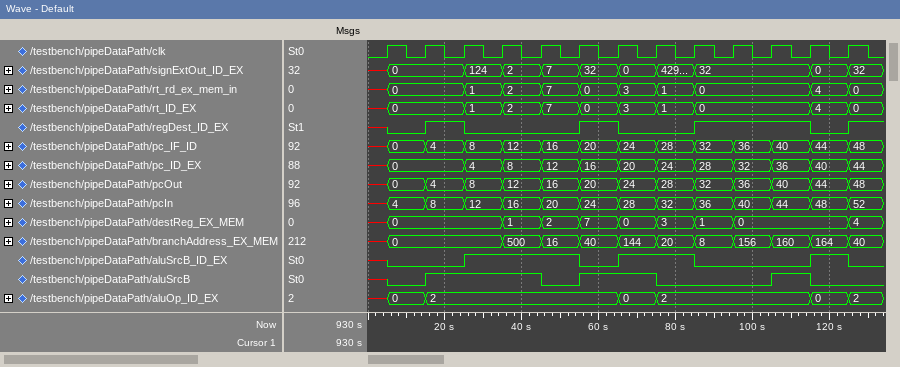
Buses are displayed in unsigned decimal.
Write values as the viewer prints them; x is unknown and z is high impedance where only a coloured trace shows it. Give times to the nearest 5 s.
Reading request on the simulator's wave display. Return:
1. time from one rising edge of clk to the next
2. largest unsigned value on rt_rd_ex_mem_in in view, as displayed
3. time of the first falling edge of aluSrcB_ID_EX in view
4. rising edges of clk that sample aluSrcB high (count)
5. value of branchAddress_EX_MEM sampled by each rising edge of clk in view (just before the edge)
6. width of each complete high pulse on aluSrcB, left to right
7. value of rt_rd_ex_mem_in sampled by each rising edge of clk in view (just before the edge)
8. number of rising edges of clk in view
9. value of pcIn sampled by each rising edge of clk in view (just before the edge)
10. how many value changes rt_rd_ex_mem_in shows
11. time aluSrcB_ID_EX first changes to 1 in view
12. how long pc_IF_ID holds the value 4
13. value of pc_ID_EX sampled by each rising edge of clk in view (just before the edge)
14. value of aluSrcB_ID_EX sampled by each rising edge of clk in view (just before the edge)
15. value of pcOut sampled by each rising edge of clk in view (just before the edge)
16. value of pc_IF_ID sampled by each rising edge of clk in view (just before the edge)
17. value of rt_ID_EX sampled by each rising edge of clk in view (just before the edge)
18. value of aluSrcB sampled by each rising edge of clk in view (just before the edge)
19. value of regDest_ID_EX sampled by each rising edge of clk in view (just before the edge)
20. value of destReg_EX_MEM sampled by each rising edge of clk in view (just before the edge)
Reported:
10 s
7
55 s
6
x, 0, 0, 0, 500, 16, 40, 144, 20, 8, 156, 160, 164
30 s, 20 s, 10 s
x, 0, 0, 1, 2, 7, 0, 3, 1, 0, 0, 0, 4
13
x, 4, 8, 12, 16, 20, 24, 28, 32, 36, 40, 44, 48
10
25 s
10 s
x, 0, 0, 4, 8, 12, 16, 20, 24, 28, 32, 36, 40
x 0 0 1 1 1 0 1 1 0 0 0 1
x, 0, 4, 8, 12, 16, 20, 24, 28, 32, 36, 40, 44
x, 0, 4, 8, 12, 16, 20, 24, 28, 32, 36, 40, 44
x, 0, 0, 1, 2, 7, 0, 3, 1, 0, 0, 0, 4
x 0 1 1 1 0 1 1 0 0 0 1 0
x 0 1 0 0 0 1 0 0 1 1 1 0
x, 0, 0, 0, 1, 2, 7, 0, 3, 1, 0, 0, 0
